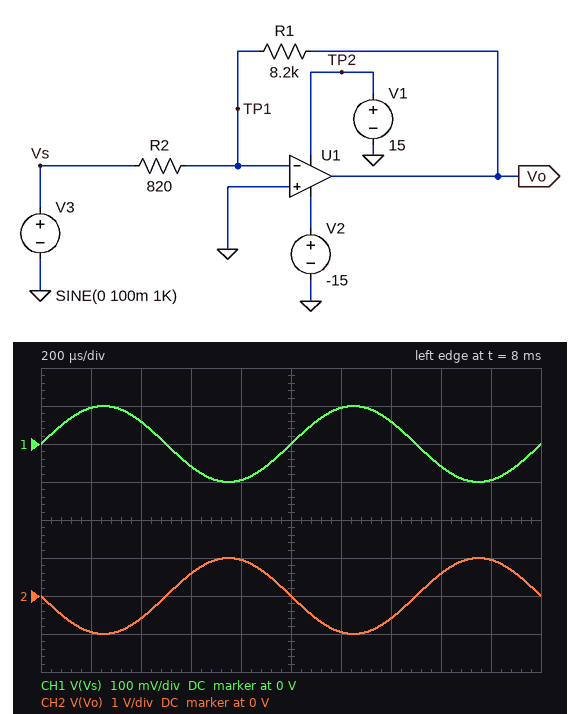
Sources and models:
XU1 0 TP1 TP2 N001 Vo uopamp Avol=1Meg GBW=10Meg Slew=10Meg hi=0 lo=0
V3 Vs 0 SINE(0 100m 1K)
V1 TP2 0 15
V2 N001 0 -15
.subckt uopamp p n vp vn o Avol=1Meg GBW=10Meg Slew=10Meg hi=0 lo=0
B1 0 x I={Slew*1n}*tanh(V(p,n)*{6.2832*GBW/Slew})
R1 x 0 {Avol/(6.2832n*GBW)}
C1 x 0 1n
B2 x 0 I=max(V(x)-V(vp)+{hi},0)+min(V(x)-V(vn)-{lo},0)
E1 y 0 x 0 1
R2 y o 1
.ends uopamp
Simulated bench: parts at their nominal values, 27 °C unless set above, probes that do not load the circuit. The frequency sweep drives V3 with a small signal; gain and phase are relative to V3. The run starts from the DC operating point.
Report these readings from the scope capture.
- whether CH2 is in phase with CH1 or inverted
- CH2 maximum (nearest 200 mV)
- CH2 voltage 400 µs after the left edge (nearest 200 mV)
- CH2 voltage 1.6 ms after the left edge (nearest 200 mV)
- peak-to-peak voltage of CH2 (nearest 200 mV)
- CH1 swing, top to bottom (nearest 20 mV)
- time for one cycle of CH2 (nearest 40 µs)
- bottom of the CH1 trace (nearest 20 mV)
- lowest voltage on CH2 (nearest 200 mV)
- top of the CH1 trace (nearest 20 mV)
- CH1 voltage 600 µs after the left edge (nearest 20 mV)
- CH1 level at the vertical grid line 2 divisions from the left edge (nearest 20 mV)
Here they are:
inverted
1.0 V
-600 mV
600 mV
2.0 V
200 mV
1.00 ms
-100 mV
-1.0 V
100 mV
-60 mV
60 mV
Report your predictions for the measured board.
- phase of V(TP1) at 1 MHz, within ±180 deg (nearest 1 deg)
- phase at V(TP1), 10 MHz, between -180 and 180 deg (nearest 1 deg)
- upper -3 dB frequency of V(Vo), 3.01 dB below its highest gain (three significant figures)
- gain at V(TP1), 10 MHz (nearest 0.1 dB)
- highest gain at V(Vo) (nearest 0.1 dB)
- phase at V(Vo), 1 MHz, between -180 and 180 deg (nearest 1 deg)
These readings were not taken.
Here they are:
42 deg
5 deg
909 kHz
-0.9 dB
20.0 dB
132 deg
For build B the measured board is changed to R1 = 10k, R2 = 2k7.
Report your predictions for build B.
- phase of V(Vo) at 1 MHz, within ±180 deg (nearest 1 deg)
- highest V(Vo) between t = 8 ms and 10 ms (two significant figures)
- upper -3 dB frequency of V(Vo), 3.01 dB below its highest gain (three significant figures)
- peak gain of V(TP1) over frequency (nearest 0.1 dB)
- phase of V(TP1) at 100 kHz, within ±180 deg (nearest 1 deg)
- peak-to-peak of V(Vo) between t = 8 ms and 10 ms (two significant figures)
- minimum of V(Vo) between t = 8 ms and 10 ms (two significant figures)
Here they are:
155 deg
370 mV
2.13 MHz
-2.1 dB
87 deg
740 mV
-370 mV
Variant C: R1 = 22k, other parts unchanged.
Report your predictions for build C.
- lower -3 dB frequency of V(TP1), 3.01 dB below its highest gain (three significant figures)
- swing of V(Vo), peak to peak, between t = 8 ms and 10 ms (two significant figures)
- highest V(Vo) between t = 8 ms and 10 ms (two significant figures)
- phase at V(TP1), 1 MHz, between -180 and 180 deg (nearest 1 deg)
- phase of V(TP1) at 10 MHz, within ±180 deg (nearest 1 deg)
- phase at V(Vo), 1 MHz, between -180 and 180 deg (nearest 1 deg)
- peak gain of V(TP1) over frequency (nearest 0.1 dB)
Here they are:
359 kHz
5.4 V
2.7 V
20 deg
2 deg
110 deg
-0.3 dB
